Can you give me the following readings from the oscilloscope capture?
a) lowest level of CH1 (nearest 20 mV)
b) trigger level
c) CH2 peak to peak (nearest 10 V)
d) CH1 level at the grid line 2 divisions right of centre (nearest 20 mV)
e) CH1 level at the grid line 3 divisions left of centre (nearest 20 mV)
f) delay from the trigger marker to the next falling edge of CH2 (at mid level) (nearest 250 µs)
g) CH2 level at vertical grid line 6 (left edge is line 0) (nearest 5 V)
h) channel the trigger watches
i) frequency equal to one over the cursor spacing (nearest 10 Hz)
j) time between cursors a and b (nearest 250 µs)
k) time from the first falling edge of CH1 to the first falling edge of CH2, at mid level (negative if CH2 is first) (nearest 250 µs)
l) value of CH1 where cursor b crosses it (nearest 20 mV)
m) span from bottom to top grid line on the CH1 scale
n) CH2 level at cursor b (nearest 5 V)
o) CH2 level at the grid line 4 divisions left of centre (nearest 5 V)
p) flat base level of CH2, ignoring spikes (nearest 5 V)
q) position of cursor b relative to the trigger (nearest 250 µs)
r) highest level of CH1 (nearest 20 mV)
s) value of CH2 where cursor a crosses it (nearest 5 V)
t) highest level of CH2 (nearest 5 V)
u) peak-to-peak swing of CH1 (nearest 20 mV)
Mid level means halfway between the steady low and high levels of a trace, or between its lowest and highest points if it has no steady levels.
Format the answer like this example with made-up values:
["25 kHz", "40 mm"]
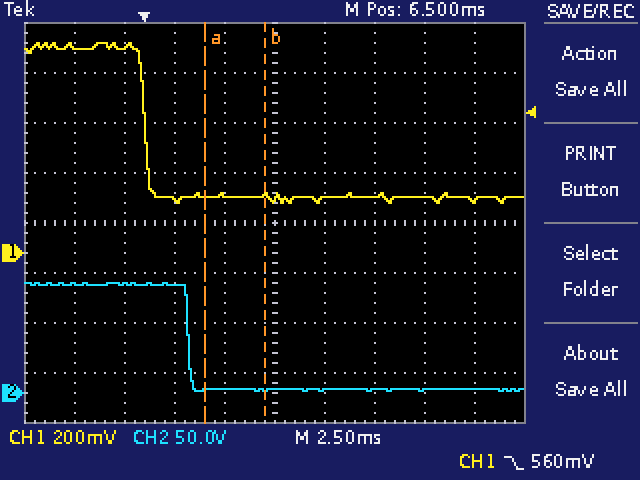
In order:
["200 mV", "560 mV", "110 V", "220 mV", "820 mV", "2.25 ms", "5 V", "CH1", "330 Hz", "3.00 ms", "+2.25 ms", "220 mV", "1.6 V", "5 V", "110 V", "5 V", "+6.00 ms", "840 mV", "5 V", "110 V", "640 mV"]
